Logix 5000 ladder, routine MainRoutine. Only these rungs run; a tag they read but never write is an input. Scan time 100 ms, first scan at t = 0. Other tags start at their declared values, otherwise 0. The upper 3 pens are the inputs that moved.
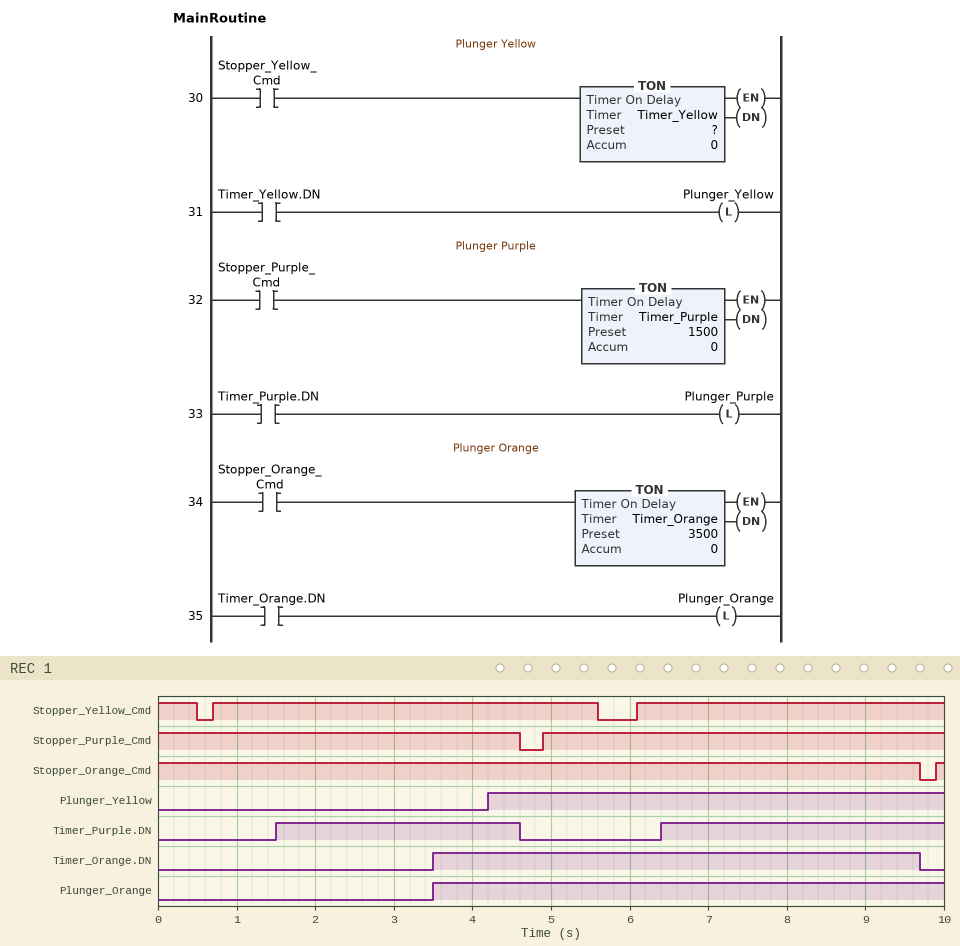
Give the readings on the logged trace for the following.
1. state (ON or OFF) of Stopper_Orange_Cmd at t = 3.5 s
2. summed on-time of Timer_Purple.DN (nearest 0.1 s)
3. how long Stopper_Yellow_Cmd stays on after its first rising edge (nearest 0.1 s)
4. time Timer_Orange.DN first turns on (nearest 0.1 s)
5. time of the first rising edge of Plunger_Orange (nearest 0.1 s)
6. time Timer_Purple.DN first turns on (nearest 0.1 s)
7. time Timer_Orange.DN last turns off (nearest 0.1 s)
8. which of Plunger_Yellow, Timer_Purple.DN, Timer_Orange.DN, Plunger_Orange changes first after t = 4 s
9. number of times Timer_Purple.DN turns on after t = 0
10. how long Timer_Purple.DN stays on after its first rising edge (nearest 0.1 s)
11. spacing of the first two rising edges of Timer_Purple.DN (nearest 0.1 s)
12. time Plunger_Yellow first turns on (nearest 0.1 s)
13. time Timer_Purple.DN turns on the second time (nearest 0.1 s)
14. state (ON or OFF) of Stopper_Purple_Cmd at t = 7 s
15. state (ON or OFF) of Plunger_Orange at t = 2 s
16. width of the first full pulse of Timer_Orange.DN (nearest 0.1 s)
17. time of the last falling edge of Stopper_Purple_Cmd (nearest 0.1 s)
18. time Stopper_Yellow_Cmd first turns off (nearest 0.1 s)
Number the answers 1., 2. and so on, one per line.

1. ON
2. 6.7 s
3. 4.9 s
4. 3.5 s
5. 3.5 s
6. 1.5 s
7. 9.7 s
8. Plunger_Yellow
9. 2
10. 3.1 s
11. 4.9 s
12. 4.2 s
13. 6.4 s
14. ON
15. OFF
16. 6.2 s
17. 4.6 s
18. 0.5 s
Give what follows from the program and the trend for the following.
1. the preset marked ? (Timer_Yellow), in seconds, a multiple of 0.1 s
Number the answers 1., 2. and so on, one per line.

1. 3.5 s
